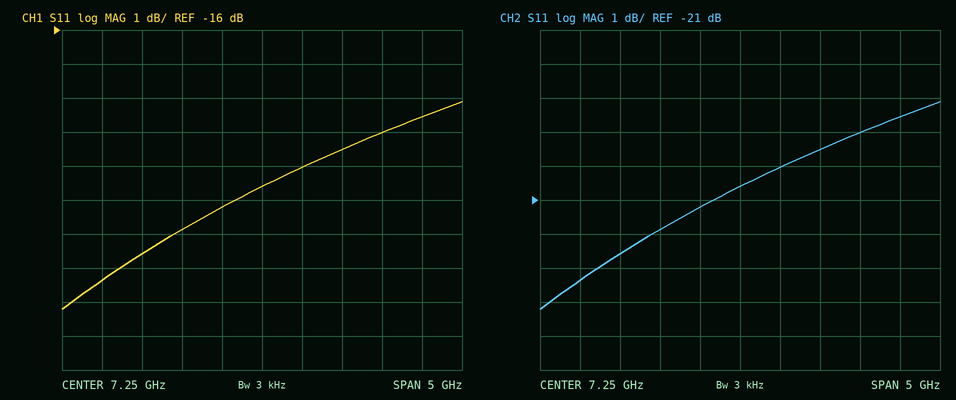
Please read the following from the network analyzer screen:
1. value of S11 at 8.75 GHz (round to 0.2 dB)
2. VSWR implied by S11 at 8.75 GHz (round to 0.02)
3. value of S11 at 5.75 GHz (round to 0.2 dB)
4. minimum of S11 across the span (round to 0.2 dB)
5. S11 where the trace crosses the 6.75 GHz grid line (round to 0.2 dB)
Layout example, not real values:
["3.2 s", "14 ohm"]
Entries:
["-19.0 dB", "1.26", "-22.6 dB", "-24.2 dB", "-21.2 dB"]
